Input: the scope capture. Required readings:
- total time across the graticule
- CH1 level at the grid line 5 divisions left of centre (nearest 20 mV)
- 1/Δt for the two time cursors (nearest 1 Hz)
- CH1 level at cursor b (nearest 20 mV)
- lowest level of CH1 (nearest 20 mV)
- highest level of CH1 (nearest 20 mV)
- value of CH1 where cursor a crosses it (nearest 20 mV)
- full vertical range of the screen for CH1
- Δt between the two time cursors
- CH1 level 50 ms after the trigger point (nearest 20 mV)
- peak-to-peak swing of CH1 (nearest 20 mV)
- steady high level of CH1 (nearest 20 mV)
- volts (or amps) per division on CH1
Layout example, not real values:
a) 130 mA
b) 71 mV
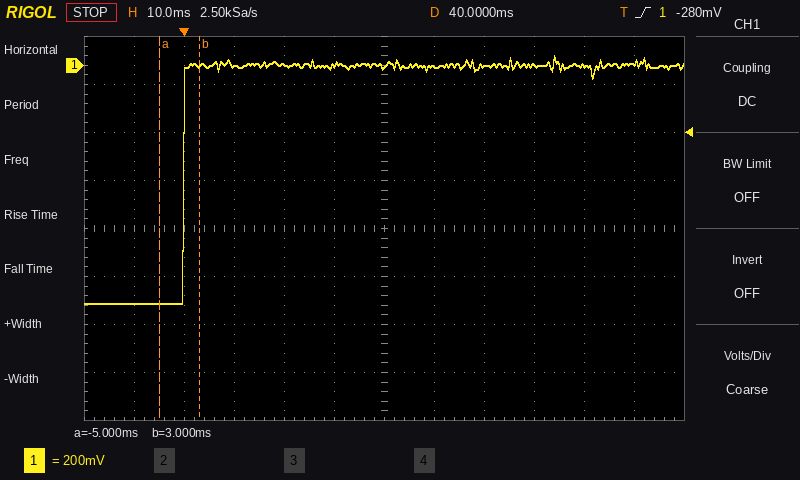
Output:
a) 120 ms
b) -1.00 V
c) 125 Hz
d) 0 mV
e) -1.00 V
f) 40 mV
g) -1.00 V
h) 1.6 V
i) 8 ms
j) 0 mV
k) 1.04 V
l) 0 mV
m) 200 mV
